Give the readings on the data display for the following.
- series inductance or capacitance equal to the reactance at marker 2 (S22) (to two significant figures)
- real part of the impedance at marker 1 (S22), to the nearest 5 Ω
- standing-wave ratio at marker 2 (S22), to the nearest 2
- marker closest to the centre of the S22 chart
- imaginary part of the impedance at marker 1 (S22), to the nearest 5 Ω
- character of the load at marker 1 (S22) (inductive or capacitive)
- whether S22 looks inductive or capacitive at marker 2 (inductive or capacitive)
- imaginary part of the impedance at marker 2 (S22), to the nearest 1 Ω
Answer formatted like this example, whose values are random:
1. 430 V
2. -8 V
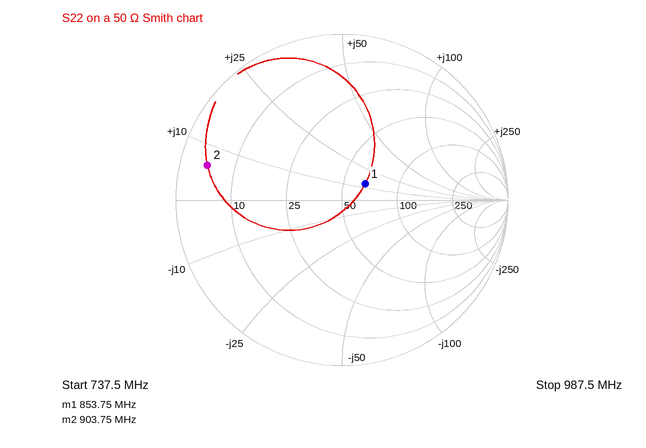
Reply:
1. 1.1 nH
2. 65 Ω
3. 12
4. marker 1
5. +15 Ω
6. inductive
7. inductive
8. +6 Ω
